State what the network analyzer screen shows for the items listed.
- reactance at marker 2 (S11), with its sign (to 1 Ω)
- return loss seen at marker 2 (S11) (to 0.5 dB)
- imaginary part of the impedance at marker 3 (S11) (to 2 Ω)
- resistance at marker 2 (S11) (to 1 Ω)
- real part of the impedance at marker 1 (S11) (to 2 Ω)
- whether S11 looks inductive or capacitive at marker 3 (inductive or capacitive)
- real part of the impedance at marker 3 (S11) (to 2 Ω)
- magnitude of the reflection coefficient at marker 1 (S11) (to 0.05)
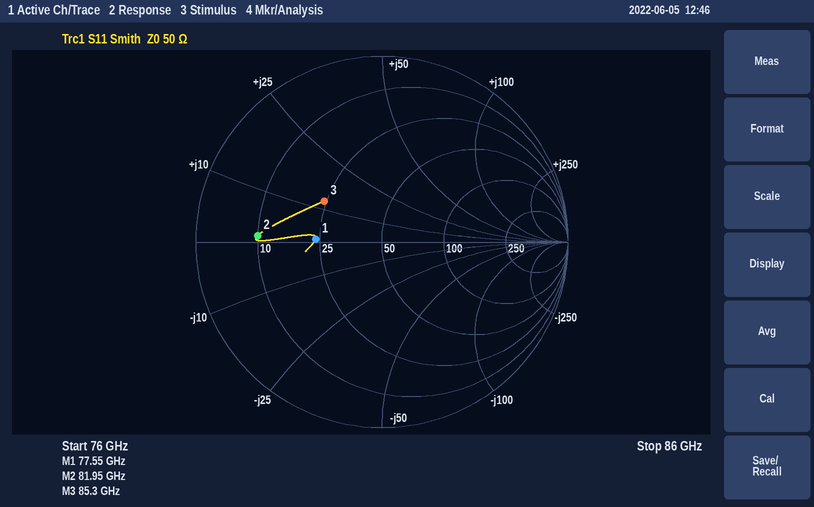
+1 Ω
3.5 dB
+12 Ω
10 Ω
24 Ω
inductive
24 Ω
0.35
